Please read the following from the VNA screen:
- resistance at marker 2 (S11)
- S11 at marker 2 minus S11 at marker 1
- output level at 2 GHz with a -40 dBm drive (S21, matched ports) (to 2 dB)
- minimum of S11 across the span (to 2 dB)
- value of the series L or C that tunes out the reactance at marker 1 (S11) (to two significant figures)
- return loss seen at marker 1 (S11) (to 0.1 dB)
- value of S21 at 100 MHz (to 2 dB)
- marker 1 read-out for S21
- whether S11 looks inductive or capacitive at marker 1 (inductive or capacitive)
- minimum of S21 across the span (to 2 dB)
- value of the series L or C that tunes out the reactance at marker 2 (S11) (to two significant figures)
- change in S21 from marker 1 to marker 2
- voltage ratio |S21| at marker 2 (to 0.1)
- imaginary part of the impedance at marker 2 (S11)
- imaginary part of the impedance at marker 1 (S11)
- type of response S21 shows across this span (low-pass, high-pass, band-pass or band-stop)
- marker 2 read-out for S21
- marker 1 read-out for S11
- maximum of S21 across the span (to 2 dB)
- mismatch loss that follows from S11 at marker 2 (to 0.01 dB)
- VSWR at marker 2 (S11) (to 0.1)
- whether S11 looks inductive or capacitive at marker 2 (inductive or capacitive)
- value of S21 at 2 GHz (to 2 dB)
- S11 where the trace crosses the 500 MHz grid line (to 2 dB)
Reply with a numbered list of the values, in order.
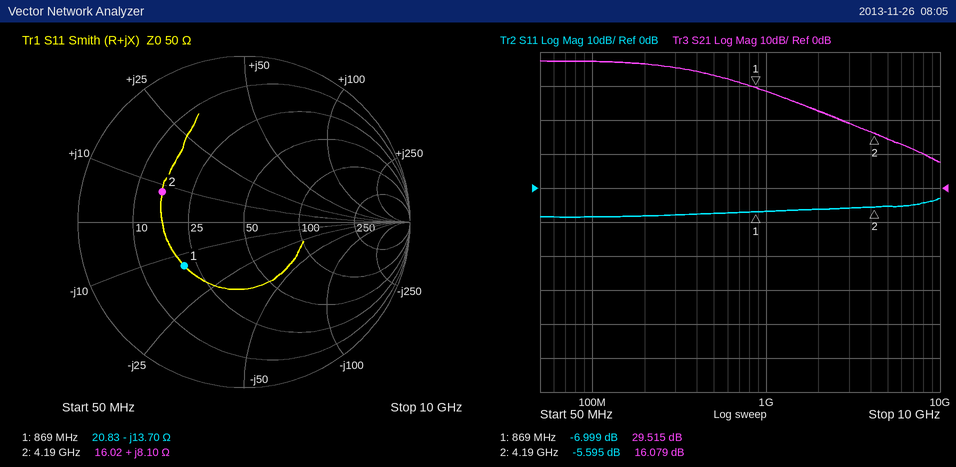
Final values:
1. 16.02 Ω
2. 1.404 dB
3. -18 dBm
4. -8 dB
5. 2.5 nH
6. 7.0 dB
7. 38 dB
8. 29.515 dB
9. capacitive
10. 8 dB
11. 4.7 pF
12. -13.436 dB
13. 6.4
14. +8.10 Ω
15. -13.70 Ω
16. low-pass
17. 16.079 dB
18. -6.999 dB
19. 38 dB
20. 1.40 dB
21. 3.2
22. inductive
23. 22 dB
24. -8 dB
